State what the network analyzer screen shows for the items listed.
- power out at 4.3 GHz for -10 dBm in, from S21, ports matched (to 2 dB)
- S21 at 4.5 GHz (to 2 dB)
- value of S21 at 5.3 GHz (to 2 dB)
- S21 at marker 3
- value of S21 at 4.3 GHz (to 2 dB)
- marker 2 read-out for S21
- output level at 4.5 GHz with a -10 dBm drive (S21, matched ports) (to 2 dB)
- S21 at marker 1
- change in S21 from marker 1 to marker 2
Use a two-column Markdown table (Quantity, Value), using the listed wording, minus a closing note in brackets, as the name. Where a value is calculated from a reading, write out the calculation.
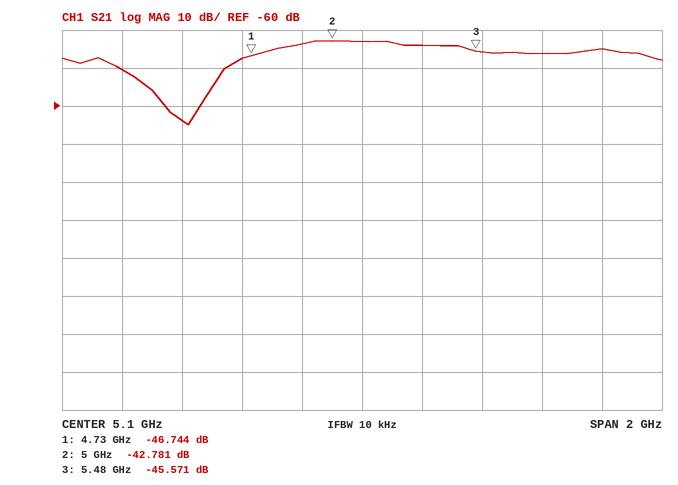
| Quantity | Value |
|---|---|
| power out at 4.3 GHz for -10 dBm in, from S21, ports matched | -10 dBm + (-50 dB) = -60 dBm |
| S21 at 4.5 GHz | -64 dB |
| value of S21 at 5.3 GHz | -44 dB |
| S21 at marker 3 | -45.571 dB |
| value of S21 at 4.3 GHz | -50 dB |
| marker 2 read-out for S21 | -42.781 dB |
| output level at 4.5 GHz with a -10 dBm drive (S21, matched ports) | -10 dBm + (-64 dB) = -74 dBm |
| S21 at marker 1 | -46.744 dB |
| change in S21 from marker 1 to marker 2 | -42.781 − (-46.744) = 3.963 dB |
